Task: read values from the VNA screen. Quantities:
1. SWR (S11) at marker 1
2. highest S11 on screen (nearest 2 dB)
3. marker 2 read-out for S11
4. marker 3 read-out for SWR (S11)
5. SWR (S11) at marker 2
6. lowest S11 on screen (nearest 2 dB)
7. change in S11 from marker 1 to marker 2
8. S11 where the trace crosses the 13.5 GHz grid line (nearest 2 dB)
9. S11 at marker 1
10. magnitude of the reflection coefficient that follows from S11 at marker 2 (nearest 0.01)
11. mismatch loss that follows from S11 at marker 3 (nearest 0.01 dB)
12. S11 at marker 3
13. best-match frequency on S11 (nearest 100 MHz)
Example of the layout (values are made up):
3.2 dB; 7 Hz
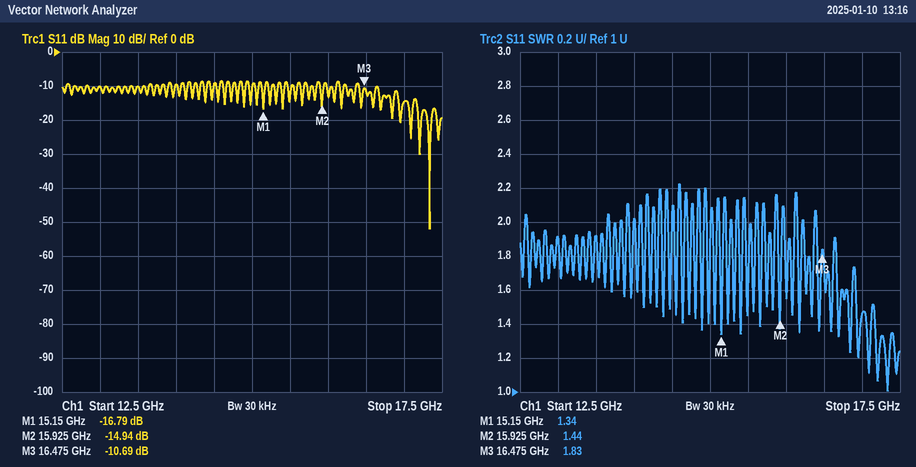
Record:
1.34; -8 dB; -14.94 dB; 1.83; 1.44; -52 dB; 1.85 dB; -10 dB; -16.79 dB; 0.18; 0.39 dB; -10.69 dB; 17.3 GHz
